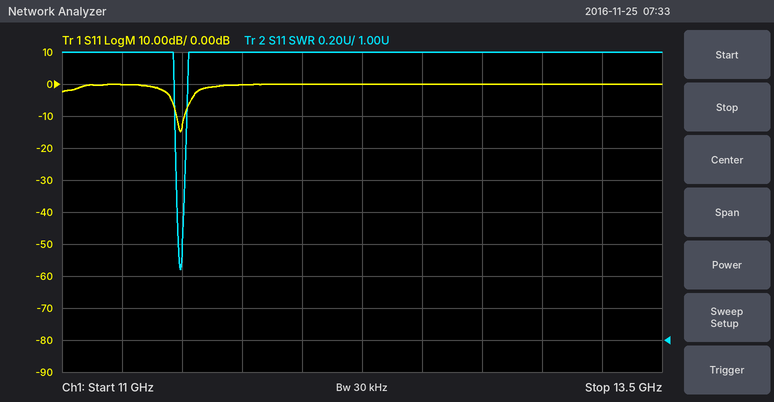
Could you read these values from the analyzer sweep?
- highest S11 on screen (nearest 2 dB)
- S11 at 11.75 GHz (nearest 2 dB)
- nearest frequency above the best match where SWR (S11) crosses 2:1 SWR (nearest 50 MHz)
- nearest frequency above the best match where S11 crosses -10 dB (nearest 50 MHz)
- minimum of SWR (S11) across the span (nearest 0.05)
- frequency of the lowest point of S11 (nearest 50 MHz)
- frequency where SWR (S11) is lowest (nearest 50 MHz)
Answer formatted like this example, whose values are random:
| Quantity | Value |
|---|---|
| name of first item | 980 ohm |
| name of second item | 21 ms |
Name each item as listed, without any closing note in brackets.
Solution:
| Quantity | Value |
|---|---|
| highest S11 on screen | 0 dB |
| S11 at 11.75 GHz | 0 dB |
| nearest frequency above the best match where SWR (S11) crosses 2:1 SWR | 11.50 GHz |
| nearest frequency above the best match where S11 crosses -10 dB | 11.50 GHz |
| minimum of SWR (S11) across the span | 1.45 |
| frequency of the lowest point of S11 | 11.50 GHz |
| frequency where SWR (S11) is lowest | 11.50 GHz |
